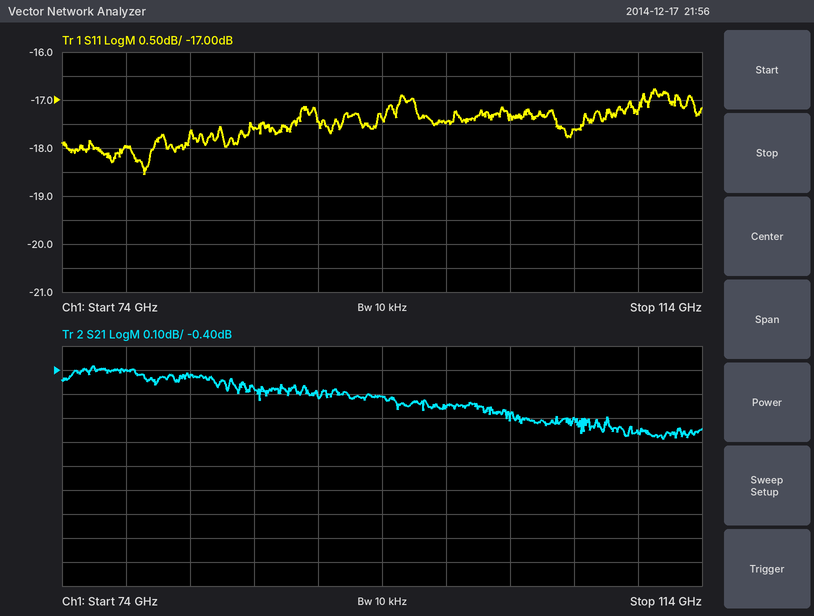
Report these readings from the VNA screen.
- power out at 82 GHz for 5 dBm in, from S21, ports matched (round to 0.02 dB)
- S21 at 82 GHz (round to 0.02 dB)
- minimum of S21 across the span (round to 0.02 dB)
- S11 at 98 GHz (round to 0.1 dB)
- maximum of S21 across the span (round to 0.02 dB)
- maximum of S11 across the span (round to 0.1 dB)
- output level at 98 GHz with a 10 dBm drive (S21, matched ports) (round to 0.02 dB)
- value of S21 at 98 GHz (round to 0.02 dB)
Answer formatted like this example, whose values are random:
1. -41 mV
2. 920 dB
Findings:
1. 4.58 dBm
2. -0.42 dB
3. -0.68 dB
4. -17.5 dB
5. -0.38 dB
6. -16.8 dB
7. 9.44 dBm
8. -0.56 dB
